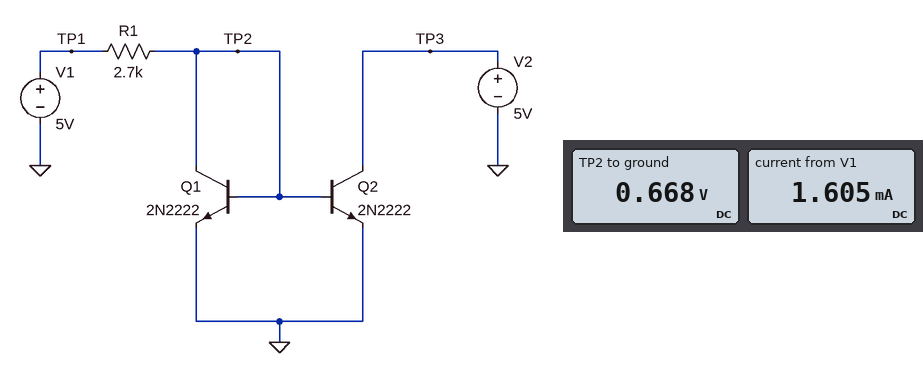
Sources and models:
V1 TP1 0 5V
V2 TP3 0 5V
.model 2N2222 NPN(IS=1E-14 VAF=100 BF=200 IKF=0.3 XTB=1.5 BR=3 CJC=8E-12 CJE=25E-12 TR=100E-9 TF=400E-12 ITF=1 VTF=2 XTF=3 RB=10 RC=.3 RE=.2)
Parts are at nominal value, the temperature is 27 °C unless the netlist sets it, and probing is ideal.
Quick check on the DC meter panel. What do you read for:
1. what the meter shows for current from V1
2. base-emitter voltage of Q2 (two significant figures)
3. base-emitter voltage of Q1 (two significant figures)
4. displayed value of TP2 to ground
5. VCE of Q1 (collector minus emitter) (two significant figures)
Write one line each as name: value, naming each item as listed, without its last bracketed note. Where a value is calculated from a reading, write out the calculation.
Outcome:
what the meter shows for current from V1: 1.605 mA
base-emitter voltage of Q2: 668 mV = 670 mV
base-emitter voltage of Q1: 668 mV = 670 mV
displayed value of TP2 to ground: 0.668 V
VCE of Q1 (collector minus emitter): 668 mV = 670 mV
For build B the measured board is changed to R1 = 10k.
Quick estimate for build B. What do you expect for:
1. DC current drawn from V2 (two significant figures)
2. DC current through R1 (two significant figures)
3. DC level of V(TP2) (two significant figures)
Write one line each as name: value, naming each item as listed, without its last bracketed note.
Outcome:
DC current drawn from V2: 450 µA
DC current through R1: 440 µA
DC level of V(TP2): 630 mV
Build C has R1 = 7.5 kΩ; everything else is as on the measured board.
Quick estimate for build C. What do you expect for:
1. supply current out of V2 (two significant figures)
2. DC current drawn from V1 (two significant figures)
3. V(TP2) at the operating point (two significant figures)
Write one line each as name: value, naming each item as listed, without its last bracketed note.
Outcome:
supply current out of V2: 600 µA
DC current drawn from V1: 580 µA
V(TP2) at the operating point: 640 mV
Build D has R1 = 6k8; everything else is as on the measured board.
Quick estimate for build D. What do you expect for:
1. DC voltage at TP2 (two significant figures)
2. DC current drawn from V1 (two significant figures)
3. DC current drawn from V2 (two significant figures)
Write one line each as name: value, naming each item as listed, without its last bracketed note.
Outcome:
DC voltage at TP2: 640 mV
DC current drawn from V1: 640 µA
DC current drawn from V2: 660 µA
